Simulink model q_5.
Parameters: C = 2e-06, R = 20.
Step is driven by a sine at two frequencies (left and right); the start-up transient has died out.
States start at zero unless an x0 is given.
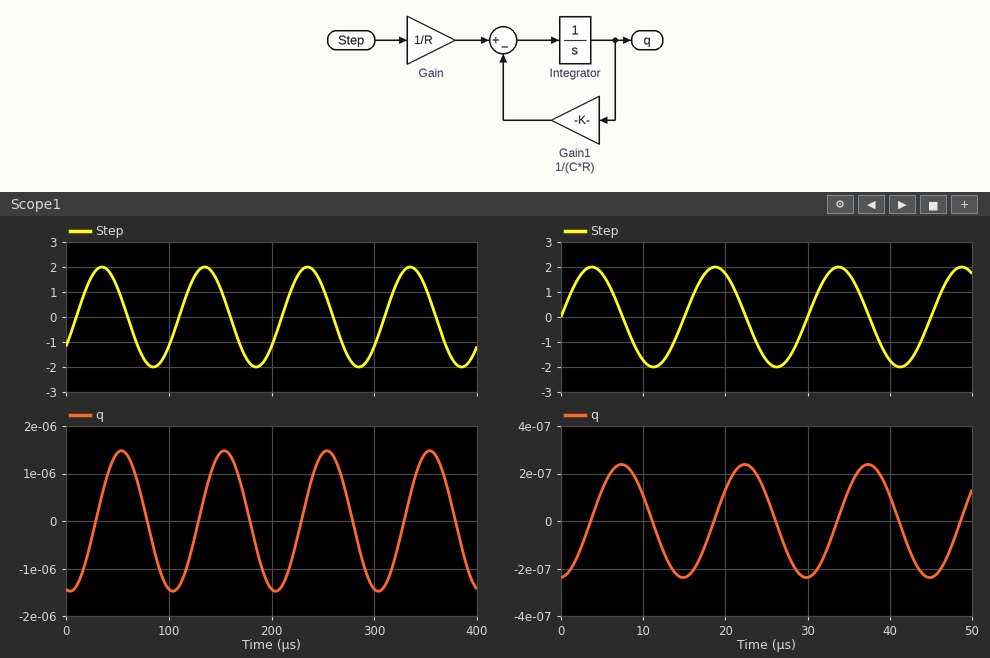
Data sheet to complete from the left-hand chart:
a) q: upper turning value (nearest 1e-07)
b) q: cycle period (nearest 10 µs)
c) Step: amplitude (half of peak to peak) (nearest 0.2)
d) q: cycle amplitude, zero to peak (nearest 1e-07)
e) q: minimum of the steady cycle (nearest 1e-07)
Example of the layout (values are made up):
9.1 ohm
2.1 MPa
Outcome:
0.0000015
100 µs
2.0
0.0000015
-0.0000015
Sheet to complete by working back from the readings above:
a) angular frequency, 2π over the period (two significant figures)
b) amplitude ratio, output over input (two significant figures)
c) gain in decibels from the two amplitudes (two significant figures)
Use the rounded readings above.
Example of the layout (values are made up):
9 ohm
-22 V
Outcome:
0.063 rad/µs
0.00000075
-120 dB
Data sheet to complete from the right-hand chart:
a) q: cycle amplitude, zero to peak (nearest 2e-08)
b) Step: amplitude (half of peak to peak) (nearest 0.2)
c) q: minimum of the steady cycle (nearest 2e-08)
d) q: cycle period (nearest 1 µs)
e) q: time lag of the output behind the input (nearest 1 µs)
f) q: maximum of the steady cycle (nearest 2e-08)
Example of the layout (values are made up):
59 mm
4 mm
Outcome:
0.00000024
2.0
-0.00000024
15 µs
4 µs
0.00000024
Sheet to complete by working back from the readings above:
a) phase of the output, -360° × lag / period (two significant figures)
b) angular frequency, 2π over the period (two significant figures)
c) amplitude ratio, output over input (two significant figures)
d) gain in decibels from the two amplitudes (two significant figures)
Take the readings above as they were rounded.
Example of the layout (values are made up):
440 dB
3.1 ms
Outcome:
-96°
0.42 rad/µs
0.00000012
-140 dB
